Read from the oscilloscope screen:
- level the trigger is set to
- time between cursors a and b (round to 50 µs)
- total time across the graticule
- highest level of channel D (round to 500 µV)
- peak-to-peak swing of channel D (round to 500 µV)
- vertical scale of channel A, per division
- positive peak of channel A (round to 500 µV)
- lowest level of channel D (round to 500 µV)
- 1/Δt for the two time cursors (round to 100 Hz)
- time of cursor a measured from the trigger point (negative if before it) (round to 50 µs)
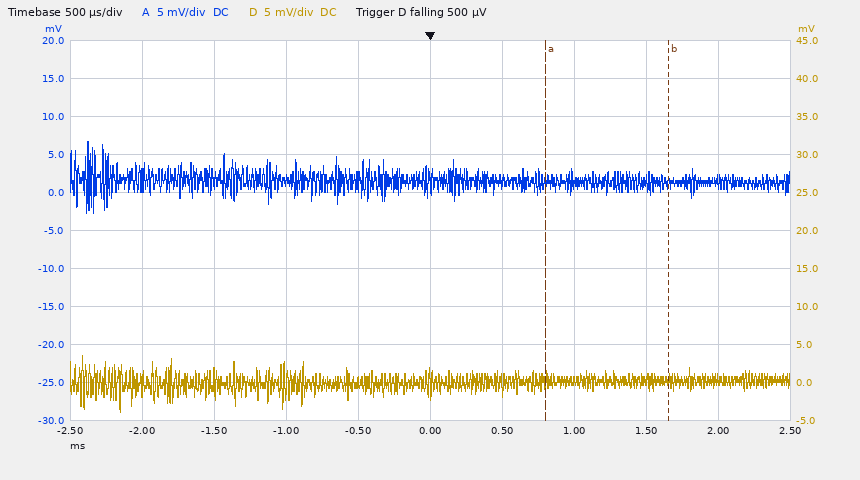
500 µV
850 µs
5 ms
3.5 mV
7.5 mV
5 mV
6.5 mV
-4.0 mV
1.2 kHz
+800 µs
